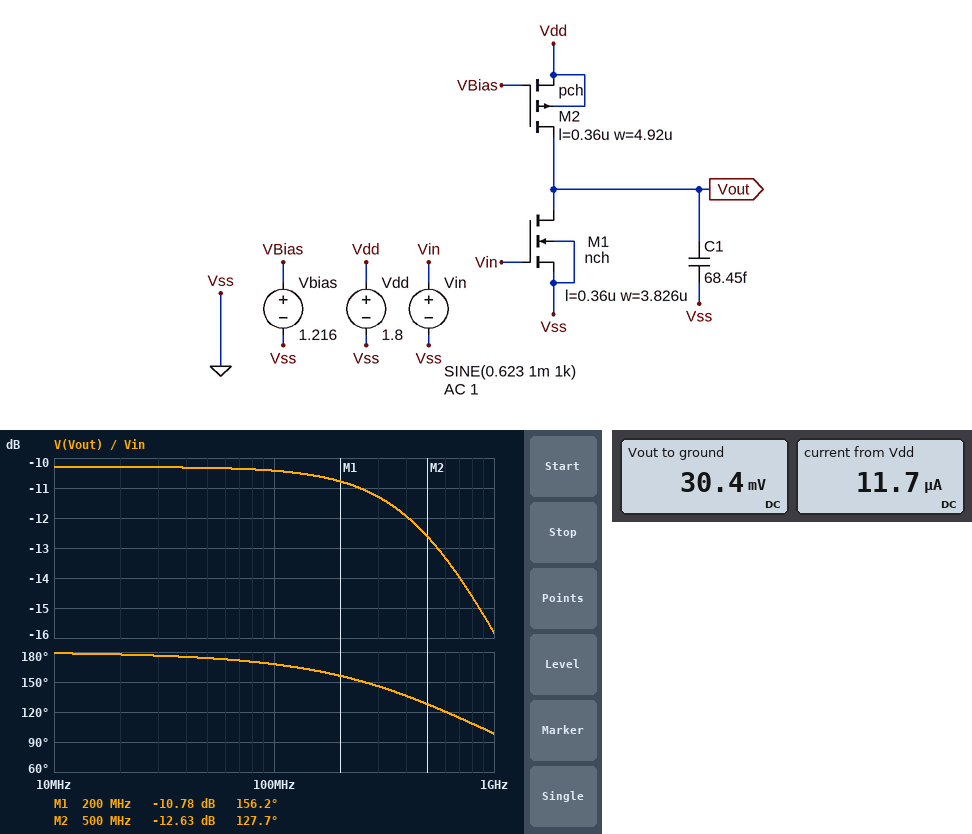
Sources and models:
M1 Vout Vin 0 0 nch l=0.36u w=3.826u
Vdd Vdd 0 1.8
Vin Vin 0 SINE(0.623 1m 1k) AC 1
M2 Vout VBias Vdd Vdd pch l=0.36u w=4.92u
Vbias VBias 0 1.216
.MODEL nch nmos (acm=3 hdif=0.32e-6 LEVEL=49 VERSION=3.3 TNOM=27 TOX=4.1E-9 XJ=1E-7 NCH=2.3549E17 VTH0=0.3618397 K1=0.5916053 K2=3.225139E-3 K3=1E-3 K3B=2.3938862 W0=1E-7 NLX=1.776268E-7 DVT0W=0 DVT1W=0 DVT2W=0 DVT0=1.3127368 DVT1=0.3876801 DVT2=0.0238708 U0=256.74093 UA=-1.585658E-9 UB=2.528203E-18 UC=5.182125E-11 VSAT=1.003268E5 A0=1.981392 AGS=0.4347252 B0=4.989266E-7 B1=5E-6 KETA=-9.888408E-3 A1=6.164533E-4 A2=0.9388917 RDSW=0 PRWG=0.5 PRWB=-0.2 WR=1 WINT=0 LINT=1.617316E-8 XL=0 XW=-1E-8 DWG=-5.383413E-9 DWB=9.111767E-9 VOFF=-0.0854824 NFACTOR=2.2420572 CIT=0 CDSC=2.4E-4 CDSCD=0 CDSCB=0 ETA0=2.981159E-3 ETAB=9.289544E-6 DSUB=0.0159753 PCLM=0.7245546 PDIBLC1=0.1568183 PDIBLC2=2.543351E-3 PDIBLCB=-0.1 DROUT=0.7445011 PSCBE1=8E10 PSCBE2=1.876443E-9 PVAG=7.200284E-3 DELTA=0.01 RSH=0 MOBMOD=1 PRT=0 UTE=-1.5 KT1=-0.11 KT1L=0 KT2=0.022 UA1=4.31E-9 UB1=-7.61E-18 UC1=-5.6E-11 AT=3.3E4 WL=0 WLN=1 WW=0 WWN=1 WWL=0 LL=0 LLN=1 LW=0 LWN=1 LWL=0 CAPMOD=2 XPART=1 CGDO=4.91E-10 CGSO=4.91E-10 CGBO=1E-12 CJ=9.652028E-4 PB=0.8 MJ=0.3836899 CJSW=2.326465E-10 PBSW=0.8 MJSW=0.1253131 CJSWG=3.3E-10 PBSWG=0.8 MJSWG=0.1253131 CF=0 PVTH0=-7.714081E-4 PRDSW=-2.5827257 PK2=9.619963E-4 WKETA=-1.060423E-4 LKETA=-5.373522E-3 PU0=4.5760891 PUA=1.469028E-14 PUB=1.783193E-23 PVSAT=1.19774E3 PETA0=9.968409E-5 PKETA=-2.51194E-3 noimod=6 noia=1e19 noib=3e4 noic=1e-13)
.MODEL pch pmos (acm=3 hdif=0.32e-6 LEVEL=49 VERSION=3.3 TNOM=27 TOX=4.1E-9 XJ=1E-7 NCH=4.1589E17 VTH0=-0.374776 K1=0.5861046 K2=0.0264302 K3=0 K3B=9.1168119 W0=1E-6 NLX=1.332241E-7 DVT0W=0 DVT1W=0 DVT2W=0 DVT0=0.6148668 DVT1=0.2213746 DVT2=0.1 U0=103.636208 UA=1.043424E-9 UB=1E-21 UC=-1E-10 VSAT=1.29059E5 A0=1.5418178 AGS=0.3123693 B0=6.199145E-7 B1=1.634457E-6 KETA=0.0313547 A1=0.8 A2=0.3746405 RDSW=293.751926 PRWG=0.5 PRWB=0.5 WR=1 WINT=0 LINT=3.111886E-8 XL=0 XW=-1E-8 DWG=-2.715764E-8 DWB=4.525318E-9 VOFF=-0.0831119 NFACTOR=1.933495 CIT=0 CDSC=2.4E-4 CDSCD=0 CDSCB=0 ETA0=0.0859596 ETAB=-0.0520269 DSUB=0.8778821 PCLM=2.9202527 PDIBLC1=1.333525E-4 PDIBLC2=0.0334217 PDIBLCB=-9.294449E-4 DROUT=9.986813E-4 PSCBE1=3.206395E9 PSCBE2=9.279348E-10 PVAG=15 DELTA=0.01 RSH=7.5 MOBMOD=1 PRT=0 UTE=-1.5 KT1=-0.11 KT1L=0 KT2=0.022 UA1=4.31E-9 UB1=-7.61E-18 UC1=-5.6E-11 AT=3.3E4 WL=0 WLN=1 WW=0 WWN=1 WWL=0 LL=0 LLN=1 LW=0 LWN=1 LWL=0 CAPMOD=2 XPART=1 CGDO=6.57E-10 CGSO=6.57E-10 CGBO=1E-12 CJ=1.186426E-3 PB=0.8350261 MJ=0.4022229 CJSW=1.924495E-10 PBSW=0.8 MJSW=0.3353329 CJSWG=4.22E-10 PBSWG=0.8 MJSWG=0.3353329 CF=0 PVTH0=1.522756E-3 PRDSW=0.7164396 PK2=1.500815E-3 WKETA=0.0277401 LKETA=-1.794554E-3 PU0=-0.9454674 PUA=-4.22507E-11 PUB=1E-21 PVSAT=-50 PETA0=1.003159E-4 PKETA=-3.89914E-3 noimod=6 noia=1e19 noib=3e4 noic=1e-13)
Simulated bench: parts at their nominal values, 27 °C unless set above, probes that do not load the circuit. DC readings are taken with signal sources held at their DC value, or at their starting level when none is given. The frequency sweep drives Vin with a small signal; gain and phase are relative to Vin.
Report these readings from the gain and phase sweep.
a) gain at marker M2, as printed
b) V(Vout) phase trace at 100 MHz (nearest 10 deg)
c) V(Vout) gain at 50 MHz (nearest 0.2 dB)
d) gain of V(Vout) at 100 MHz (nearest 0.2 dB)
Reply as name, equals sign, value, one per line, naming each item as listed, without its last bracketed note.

gain at marker M2, as printed = -12.63 dB
V(Vout) phase trace at 100 MHz = 170 deg
V(Vout) gain at 50 MHz = -10.4 dB
gain of V(Vout) at 100 MHz = -10.4 dB
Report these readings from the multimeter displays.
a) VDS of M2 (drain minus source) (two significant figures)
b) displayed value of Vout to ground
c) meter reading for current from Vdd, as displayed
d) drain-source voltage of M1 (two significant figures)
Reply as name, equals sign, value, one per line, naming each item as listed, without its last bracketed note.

VDS of M2 (drain minus source) = -1.8 V
displayed value of Vout to ground = 30.4 mV
meter reading for current from Vdd, as displayed = 11.7 µA
drain-source voltage of M1 = 30 mV
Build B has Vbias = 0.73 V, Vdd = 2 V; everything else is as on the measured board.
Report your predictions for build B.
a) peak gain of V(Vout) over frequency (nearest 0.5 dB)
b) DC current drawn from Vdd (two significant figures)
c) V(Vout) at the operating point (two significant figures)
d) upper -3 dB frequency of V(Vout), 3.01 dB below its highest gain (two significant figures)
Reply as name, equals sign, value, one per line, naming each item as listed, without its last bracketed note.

peak gain of V(Vout) over frequency = -3.5 dB
DC current drawn from Vdd = 41 µA
V(Vout) at the operating point = 1.9 V
upper -3 dB frequency of V(Vout), 3.01 dB below its highest gain = 1.1 GHz
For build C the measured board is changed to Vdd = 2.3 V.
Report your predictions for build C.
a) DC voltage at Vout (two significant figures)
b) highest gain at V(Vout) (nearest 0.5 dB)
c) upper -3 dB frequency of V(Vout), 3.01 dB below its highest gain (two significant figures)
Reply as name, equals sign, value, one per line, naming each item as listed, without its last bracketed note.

DC voltage at Vout = 2.2 V
highest gain at V(Vout) = -1.0 dB
upper -3 dB frequency of V(Vout), 3.01 dB below its highest gain = 850 MHz
